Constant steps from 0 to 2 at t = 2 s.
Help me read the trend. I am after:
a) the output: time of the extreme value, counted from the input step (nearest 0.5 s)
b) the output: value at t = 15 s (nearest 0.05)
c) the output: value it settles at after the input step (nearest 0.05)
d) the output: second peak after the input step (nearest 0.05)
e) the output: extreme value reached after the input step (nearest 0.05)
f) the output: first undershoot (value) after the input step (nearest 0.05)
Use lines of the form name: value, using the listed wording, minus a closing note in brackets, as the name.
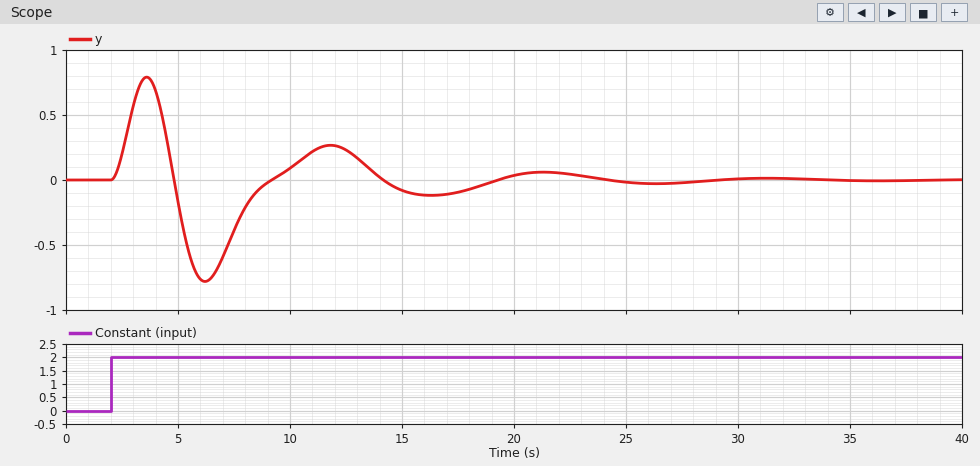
the output: time of the extreme value, counted from the input step: 1.5 s
the output: value at t = 15 s: -0.10
the output: value it settles at after the input step: 0.00
the output: second peak after the input step: 0.25
the output: extreme value reached after the input step: 0.80
the output: first undershoot (value) after the input step: -0.80
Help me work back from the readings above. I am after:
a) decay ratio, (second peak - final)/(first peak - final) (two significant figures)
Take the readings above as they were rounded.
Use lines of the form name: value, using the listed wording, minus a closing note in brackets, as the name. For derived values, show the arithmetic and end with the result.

decay ratio, (second peak - final)/(first peak - final): (0.25 - 0) / (0.8 - 0) = 0.31
